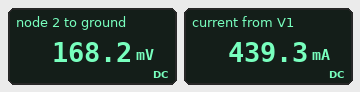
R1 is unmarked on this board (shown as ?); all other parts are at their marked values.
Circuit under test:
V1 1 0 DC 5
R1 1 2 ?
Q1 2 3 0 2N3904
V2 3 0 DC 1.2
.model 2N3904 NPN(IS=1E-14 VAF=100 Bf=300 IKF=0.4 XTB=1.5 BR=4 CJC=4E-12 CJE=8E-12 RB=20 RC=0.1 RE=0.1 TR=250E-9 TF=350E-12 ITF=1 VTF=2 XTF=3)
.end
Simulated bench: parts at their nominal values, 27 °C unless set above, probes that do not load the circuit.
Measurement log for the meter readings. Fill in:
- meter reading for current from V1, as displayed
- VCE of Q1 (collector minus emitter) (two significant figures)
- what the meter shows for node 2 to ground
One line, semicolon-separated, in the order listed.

439.3 mA; 170 mV; 168.2 mV
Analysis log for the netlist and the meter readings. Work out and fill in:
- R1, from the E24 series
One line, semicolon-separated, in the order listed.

11 Ω
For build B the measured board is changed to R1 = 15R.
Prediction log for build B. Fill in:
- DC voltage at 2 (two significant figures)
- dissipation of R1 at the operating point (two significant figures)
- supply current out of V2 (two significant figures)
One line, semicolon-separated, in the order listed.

130 mV; 1.6 W; 17 mA
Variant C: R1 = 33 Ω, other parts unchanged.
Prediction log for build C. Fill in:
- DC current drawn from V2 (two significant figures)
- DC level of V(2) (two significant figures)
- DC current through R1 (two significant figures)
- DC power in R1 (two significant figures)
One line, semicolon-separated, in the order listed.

19 mA; 71 mV; 150 mA; 740 mW
